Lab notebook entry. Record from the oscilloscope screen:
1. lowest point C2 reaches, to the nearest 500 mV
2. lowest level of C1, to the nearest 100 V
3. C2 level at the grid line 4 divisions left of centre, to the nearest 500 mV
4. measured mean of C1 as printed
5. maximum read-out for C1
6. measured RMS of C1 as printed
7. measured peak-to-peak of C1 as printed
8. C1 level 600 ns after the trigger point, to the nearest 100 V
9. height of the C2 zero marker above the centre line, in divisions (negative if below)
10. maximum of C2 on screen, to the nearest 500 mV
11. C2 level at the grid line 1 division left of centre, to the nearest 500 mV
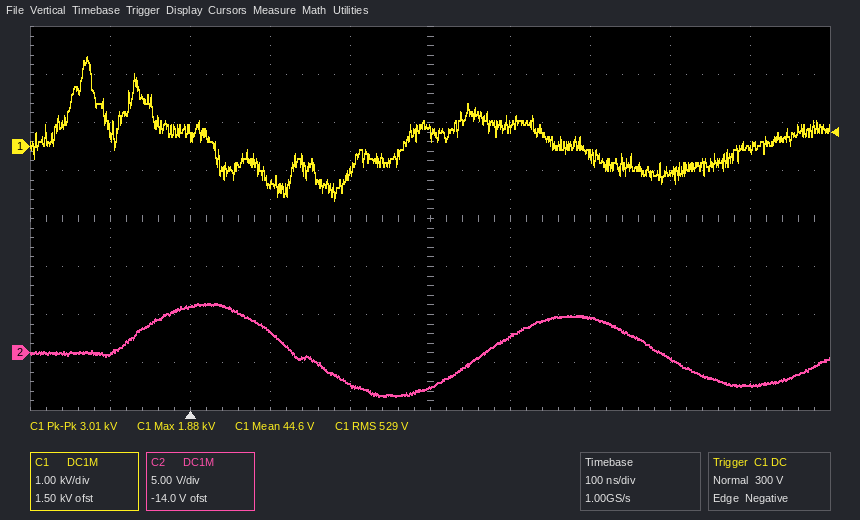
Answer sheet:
-4.5 V
-1.1 kV
0.0 V
44.6 V
1.88 kV
529 V
3.01 kV
-500 V
-2.8 div
5.0 V
-3.5 V
